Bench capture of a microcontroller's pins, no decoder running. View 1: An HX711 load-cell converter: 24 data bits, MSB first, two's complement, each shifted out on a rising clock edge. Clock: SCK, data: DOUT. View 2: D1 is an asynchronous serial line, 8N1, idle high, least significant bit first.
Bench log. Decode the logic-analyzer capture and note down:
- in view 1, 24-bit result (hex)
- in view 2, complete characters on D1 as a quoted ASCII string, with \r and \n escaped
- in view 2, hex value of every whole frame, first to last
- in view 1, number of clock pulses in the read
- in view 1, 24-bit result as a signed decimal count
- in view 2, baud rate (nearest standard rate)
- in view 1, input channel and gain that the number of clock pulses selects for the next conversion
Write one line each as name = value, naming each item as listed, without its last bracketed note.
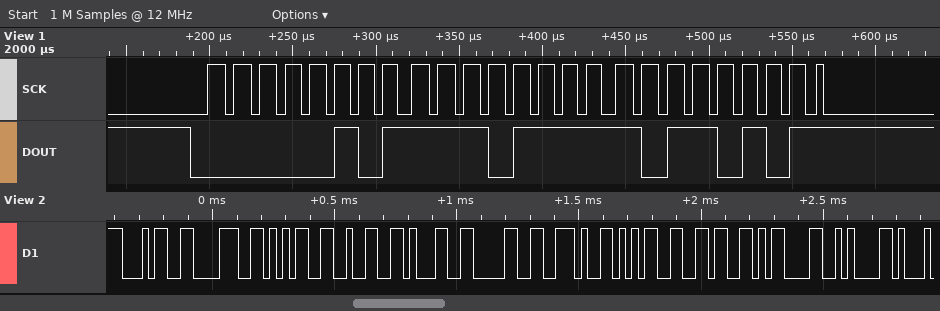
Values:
in view 1, 24-bit result = 0x05EFB5
in view 2, complete characters on D1 as a quoted ASCII string, with \r and \n escaped = "485210.56\r\n"
in view 2, hex value of every whole frame, first to last = 0x34 0x38 0x35 0x32 0x31 0x30 0x2E 0x35 0x36 0x0D 0x0A
in view 1, number of clock pulses in the read = 25
in view 1, 24-bit result as a signed decimal count = 389045
in view 2, baud rate = 38400 baud
in view 1, input channel and gain that the number of clock pulses selects for the next conversion = channel A, gain 128
